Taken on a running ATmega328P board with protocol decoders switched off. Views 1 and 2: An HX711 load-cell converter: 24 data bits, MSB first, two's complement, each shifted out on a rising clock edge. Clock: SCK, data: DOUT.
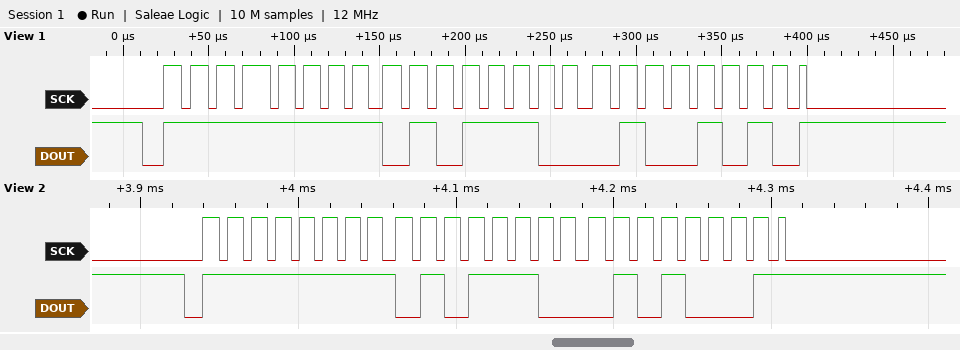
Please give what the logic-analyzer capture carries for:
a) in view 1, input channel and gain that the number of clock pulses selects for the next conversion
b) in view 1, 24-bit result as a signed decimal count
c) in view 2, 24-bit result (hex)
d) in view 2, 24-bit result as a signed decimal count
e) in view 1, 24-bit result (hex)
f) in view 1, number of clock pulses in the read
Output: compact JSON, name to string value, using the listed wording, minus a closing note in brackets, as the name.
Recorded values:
{"in view 1, input channel and gain that the number of clock pulses selects for the next conversion": "channel A, gain 128", "in view 1, 24-bit result as a signed decimal count": "-41910", "in view 2, 24-bit result": "0xFF5C51", "in view 2, 24-bit result as a signed decimal count": "-41903", "in view 1, 24-bit result": "0xFF5C4A", "in view 1, number of clock pulses in the read": "25"}
